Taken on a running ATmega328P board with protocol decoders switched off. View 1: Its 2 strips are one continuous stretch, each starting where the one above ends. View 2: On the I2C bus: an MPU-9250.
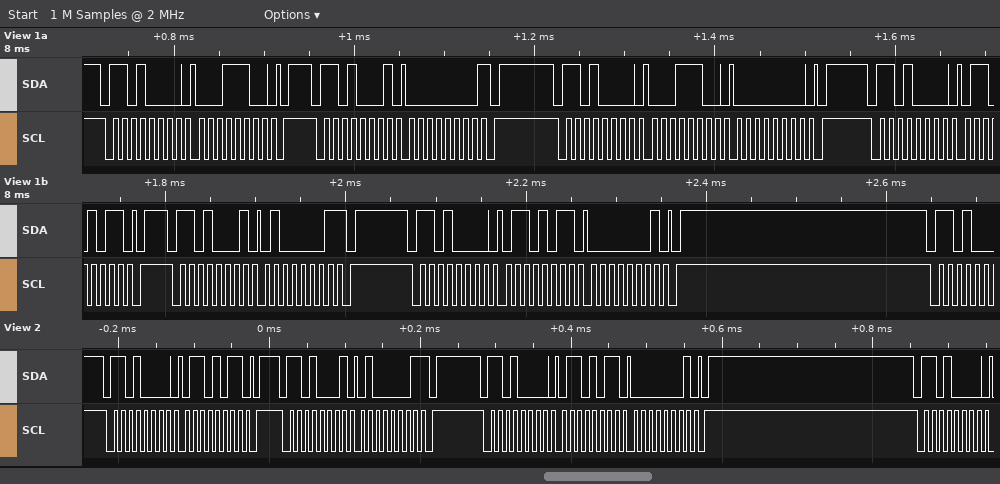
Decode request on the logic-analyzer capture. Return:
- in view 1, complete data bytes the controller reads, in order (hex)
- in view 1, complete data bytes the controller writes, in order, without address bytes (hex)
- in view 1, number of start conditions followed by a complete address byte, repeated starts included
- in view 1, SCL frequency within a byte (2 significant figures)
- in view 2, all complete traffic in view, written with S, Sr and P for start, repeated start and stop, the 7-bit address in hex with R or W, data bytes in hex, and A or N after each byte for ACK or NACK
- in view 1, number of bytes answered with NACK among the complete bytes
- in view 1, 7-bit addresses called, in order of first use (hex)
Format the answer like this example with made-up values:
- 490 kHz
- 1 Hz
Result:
- 00 41
- 1C 1C 00 6B 6B 01
- 6
- 100 kHz
- S 68W A 6B A P S 68R A 41 N P S 68W A 6B A 01 A P S 68W A
- 2
- 0x68
